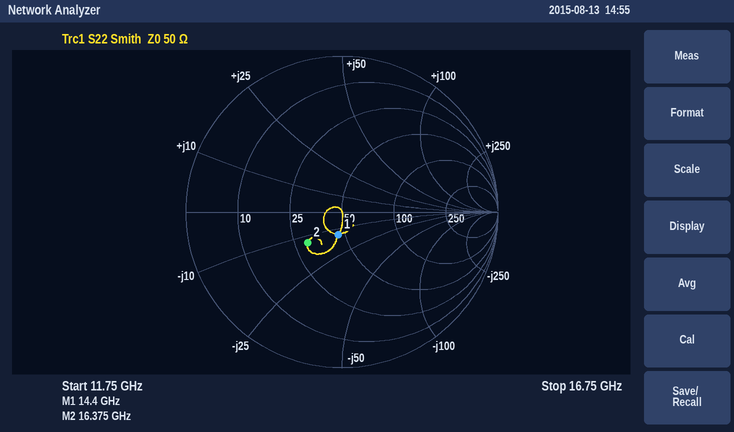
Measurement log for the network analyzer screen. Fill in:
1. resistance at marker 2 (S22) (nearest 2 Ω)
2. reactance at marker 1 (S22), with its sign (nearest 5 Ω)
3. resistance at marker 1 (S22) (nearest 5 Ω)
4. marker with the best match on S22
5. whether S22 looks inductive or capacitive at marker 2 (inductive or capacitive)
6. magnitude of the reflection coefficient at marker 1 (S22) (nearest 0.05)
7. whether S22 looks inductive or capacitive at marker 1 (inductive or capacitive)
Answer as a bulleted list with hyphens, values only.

- 30 Ω
- -15 Ω
- 45 Ω
- marker 1
- capacitive
- 0.15
- capacitive
